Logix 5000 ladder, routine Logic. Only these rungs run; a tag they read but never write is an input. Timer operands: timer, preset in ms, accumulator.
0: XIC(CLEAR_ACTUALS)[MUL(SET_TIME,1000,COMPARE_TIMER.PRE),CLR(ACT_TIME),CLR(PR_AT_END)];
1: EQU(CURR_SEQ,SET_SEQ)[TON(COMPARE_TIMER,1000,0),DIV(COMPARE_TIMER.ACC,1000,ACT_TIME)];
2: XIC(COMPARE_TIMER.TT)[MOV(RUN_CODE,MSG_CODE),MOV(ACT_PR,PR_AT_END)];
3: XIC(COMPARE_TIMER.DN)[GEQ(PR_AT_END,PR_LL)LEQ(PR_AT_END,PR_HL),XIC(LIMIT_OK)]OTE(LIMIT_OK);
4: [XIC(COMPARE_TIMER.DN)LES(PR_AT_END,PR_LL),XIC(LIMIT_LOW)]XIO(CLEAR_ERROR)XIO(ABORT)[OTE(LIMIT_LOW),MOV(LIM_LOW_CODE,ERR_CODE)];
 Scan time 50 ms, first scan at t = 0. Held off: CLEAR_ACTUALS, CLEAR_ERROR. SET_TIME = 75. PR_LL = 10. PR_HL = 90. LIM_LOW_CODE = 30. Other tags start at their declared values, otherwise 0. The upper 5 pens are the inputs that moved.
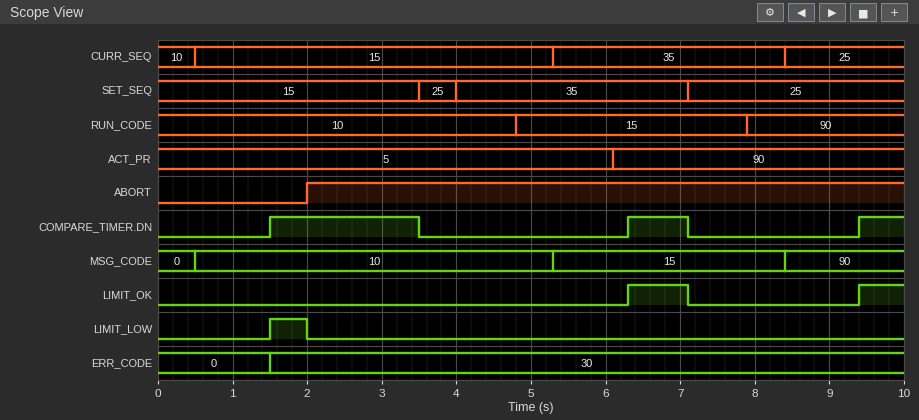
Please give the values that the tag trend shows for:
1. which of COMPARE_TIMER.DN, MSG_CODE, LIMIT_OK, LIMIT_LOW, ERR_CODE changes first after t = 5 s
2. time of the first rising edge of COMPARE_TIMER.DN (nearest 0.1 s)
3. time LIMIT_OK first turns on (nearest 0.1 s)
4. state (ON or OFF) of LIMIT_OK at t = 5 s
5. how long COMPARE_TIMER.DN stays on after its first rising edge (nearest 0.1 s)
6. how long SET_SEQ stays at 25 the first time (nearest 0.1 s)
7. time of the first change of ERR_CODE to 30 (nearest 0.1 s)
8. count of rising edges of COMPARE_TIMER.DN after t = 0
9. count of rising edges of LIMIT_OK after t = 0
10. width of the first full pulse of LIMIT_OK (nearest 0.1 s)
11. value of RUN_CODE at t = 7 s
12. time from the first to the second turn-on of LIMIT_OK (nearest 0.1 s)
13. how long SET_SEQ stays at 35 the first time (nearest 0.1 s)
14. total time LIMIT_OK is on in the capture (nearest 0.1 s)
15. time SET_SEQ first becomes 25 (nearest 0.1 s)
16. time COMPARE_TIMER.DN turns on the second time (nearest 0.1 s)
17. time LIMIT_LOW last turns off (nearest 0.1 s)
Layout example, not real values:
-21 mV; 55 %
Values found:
MSG_CODE; 1.5 s; 6.3 s; OFF; 2.0 s; 0.5 s; 1.5 s; 3; 2; 0.8 s; 15; 3.1 s; 3.1 s; 1.4 s; 3.5 s; 6.3 s; 2.0 s
